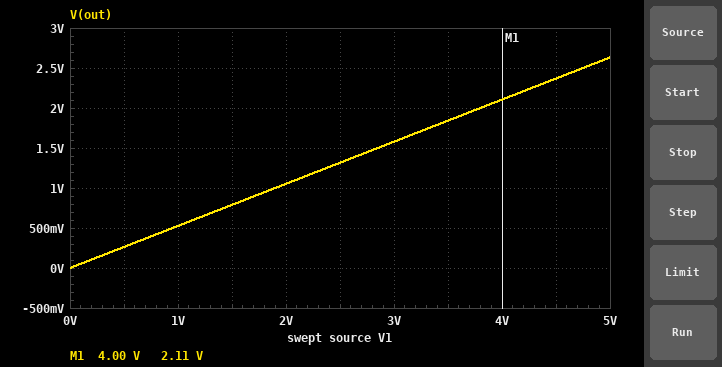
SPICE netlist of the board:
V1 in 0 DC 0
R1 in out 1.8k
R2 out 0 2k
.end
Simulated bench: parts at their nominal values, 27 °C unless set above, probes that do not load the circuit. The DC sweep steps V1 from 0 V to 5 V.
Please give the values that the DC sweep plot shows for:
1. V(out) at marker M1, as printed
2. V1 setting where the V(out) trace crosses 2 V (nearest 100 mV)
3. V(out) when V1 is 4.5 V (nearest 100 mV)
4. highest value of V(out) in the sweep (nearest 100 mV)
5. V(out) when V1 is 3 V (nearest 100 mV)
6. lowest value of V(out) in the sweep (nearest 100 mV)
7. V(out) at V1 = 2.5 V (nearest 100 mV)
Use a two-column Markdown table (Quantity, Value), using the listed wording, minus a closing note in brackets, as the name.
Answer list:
| Quantity | Value |
|---|---|
| V(out) at marker M1, as printed | 2.11 V |
| V1 setting where the V(out) trace crosses 2 V | 3.8 V |
| V(out) when V1 is 4.5 V | 2.4 V |
| highest value of V(out) in the sweep | 2.6 V |
| V(out) when V1 is 3 V | 1.6 V |
| lowest value of V(out) in the sweep | 0 V |
| V(out) at V1 = 2.5 V | 1.3 V |
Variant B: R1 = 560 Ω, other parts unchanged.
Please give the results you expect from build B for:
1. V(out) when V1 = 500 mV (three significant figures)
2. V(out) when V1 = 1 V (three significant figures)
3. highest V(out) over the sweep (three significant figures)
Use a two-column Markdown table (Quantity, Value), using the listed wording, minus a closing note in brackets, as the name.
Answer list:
| Quantity | Value |
|---|---|
| V(out) when V1 = 500 mV | 391 mV |
| V(out) when V1 = 1 V | 781 mV |
| highest V(out) over the sweep | 3.91 V |
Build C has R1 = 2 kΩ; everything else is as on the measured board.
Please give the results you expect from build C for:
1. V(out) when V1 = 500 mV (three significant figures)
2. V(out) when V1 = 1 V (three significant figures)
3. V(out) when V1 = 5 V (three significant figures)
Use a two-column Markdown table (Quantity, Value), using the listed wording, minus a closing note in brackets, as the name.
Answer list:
| Quantity | Value |
|---|---|
| V(out) when V1 = 500 mV | 250 mV |
| V(out) when V1 = 1 V | 500 mV |
| V(out) when V1 = 5 V | 2.50 V |
